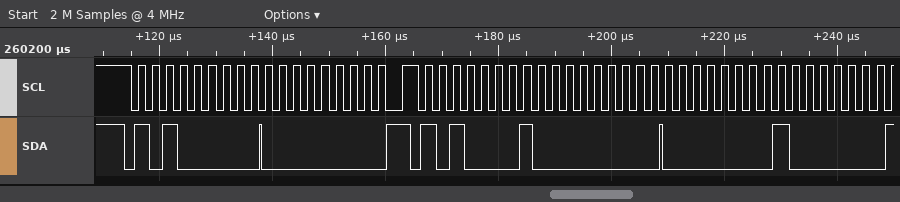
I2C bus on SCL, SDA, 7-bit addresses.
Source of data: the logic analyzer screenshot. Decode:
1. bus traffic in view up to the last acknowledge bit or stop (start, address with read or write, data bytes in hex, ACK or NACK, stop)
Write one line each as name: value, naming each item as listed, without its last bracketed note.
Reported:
bus traffic in view up to the last acknowledge bit or stop: start, address 50 write ACK, 00 ACK, repeated start, address 50 read ACK, 00 ACK, 01 ACK
